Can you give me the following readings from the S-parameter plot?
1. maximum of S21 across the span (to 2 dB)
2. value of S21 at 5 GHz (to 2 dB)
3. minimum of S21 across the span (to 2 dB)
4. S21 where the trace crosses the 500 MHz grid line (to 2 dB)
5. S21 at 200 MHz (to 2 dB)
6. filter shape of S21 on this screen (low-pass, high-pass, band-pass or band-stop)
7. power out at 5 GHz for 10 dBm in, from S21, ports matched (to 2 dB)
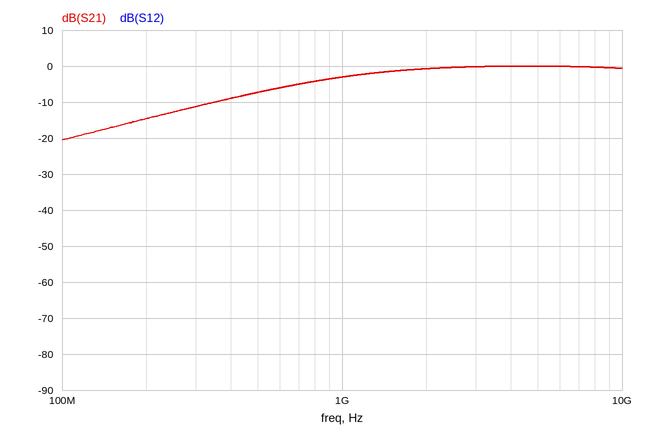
0 dB
0 dB
-20 dB
-8 dB
-14 dB
high-pass
10 dBm
